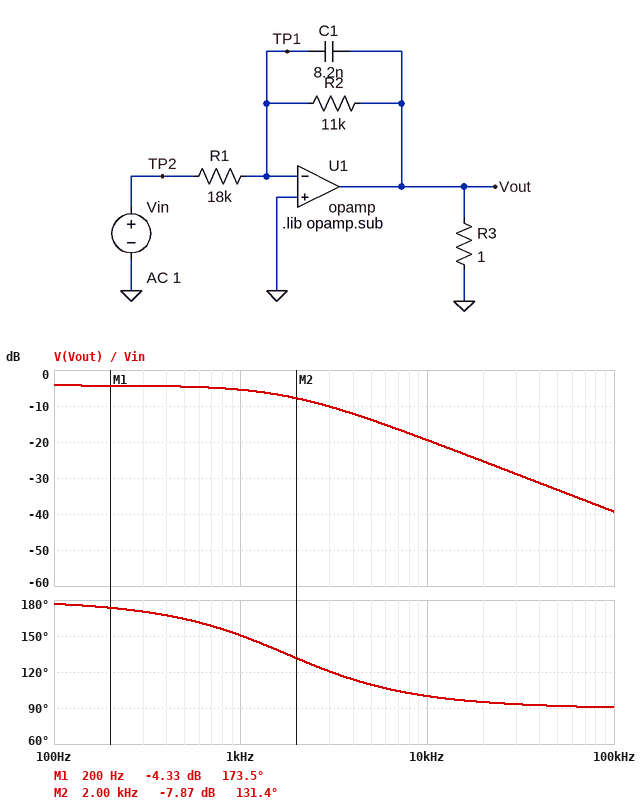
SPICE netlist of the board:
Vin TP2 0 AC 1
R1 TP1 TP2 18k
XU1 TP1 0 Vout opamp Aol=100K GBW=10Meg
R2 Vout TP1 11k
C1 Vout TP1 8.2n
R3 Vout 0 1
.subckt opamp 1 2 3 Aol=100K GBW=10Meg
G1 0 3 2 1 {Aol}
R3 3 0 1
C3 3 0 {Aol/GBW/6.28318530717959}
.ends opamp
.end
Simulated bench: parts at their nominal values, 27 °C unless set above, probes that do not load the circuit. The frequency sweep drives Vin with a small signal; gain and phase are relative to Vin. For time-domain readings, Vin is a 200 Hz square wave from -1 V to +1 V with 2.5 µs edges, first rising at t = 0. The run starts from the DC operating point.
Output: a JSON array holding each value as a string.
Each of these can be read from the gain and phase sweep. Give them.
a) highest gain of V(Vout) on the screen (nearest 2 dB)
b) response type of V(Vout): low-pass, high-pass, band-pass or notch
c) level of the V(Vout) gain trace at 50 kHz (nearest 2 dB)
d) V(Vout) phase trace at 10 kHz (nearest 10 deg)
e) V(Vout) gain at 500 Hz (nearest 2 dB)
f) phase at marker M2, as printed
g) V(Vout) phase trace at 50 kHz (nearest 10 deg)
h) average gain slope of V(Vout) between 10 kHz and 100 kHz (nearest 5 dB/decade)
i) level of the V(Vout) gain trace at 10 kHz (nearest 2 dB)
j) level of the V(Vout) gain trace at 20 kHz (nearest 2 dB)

["-4 dB", "low-pass", "-34 dB", "100 deg", "-4 dB", "131.4 deg", "90 deg", "-20 dB/decade", "-20 dB", "-26 dB"]
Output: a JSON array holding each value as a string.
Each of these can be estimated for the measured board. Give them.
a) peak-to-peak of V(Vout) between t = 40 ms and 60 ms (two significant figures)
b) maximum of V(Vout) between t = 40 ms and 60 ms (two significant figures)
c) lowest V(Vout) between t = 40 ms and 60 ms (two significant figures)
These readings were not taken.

["1.2 V", "610 mV", "-610 mV"]
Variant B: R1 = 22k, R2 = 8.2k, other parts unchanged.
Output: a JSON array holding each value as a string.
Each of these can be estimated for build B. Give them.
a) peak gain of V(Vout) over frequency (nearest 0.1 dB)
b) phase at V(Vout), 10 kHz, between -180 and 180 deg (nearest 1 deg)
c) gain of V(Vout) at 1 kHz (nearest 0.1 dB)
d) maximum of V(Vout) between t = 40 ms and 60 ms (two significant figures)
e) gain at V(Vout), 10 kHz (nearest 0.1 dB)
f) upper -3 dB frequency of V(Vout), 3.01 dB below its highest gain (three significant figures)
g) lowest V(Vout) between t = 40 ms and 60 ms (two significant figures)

["-8.6 dB", "103 deg", "-9.3 dB", "370 mV", "-21.3 dB", "2.37 kHz", "-370 mV"]
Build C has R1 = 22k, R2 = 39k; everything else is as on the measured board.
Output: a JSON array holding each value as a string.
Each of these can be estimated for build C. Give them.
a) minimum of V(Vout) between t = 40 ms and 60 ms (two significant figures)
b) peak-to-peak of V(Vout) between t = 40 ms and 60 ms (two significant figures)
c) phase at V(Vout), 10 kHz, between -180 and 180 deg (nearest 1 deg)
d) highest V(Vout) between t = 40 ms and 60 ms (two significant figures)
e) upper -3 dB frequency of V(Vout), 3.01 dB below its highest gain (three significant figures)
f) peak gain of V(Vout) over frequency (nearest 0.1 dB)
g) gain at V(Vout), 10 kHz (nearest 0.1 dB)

["-1.8 V", "3.5 V", "93 deg", "1.8 V", "498 Hz", "5.0 dB", "-21.1 dB"]
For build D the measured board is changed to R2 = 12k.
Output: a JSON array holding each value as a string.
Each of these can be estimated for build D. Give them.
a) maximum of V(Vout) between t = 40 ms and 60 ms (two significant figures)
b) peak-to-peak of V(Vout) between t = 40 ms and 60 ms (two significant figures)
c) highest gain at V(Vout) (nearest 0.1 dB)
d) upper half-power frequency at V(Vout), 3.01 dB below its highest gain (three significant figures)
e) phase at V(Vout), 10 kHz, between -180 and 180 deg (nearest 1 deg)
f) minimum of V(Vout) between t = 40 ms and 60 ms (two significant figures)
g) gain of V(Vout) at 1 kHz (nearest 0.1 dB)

["670 mV", "1.3 V", "-3.5 dB", "1.62 kHz", "99 deg", "-670 mV", "-4.9 dB"]
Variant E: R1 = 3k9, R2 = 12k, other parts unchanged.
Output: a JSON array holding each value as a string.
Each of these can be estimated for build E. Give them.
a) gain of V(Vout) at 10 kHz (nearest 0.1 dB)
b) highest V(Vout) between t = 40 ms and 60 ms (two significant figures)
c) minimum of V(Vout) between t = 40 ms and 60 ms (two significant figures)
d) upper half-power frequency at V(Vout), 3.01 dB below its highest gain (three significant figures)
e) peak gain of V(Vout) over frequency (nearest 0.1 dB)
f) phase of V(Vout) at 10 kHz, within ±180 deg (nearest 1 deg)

["-6.2 dB", "3.1 V", "-3.1 V", "1.62 kHz", "9.8 dB", "99 deg"]
